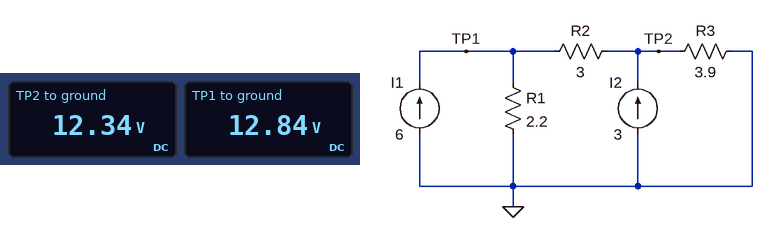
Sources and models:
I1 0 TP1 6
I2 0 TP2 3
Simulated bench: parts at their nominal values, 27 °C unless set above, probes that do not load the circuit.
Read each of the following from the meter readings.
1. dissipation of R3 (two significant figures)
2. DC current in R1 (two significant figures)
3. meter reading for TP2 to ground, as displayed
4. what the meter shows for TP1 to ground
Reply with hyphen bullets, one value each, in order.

- 39 W
- 5.8 A
- 12.34 V
- 12.84 V
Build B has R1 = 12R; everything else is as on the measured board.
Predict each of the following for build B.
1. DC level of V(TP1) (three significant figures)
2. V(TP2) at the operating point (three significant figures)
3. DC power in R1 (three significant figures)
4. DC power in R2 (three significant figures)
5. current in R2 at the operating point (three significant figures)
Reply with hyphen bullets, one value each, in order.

- 33.7 V
- 24.1 V
- 94.7 W
- 30.5 W
- 3.19 A
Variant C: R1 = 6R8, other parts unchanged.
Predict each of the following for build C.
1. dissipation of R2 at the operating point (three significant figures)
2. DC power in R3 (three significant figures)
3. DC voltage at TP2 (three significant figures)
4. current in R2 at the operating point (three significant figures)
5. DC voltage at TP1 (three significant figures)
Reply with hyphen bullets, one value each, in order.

- 13.5 W
- 102 W
- 20.0 V
- 2.12 A
- 26.4 V
